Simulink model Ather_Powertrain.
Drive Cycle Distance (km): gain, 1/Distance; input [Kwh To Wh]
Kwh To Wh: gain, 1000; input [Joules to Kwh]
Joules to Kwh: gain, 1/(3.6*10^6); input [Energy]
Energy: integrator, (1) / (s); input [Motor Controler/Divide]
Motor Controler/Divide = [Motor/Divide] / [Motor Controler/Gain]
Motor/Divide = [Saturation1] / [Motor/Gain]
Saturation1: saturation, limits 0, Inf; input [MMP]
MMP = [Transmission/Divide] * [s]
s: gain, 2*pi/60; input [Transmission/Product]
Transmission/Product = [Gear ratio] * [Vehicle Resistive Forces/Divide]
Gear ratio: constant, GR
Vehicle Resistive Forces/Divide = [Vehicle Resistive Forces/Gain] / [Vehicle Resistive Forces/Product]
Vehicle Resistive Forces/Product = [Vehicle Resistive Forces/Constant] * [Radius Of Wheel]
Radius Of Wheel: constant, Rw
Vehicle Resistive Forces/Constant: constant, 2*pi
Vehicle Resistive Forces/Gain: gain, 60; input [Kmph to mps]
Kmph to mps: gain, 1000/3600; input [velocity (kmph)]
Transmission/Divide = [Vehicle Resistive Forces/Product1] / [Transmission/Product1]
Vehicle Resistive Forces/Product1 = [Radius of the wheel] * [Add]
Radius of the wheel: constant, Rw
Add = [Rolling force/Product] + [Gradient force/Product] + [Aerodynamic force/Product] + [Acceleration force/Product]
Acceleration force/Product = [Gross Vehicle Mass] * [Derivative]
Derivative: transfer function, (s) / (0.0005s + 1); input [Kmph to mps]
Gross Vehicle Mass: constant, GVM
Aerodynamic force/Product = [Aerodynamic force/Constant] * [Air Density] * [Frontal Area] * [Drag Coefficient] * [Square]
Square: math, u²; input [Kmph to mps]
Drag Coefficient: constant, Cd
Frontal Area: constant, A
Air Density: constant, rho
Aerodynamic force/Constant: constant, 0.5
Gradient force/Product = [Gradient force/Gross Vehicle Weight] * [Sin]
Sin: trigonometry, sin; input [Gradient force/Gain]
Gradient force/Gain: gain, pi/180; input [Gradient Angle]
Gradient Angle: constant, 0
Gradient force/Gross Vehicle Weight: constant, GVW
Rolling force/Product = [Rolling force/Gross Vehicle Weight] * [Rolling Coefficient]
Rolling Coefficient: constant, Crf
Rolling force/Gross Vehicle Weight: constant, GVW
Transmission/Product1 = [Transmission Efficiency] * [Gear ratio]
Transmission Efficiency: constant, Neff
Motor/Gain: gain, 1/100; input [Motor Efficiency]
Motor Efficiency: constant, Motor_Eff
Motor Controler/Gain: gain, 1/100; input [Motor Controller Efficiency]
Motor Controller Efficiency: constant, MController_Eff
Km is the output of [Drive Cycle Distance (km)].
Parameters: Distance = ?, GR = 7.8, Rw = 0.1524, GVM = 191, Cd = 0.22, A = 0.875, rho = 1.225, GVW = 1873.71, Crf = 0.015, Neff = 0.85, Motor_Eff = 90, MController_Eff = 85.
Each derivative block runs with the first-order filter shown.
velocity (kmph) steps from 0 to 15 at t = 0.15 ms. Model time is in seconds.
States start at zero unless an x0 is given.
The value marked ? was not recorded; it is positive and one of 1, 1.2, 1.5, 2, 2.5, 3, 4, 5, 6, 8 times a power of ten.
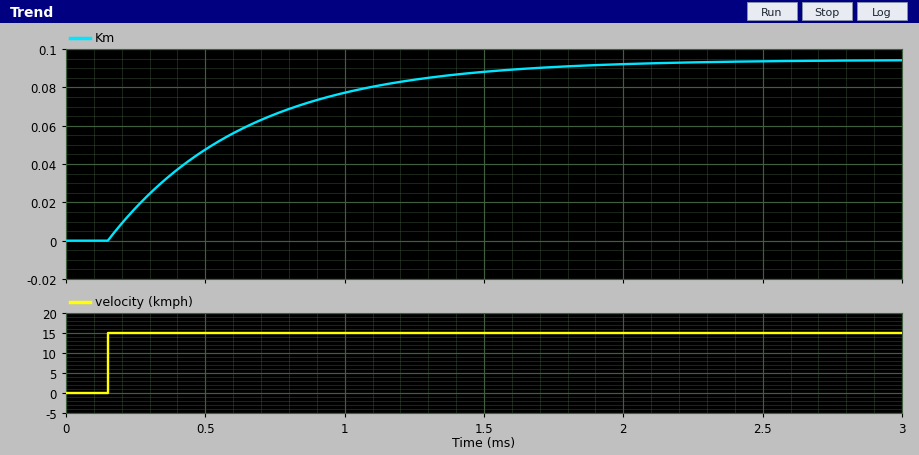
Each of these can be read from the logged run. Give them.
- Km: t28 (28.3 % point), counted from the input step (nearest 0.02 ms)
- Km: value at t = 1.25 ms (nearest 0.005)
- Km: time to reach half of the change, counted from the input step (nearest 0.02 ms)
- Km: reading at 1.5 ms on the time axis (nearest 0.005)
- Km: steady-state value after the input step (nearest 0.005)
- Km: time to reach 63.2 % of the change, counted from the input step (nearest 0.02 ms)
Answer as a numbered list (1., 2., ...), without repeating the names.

1. 0.16 ms
2. 0.085
3. 0.34 ms
4. 0.090
5. 0.095
6. 0.50 ms
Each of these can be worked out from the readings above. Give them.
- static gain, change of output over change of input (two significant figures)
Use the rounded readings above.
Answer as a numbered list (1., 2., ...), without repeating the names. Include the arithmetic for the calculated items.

1. (0.095 - 0) / (15 - 0) = 0.0063
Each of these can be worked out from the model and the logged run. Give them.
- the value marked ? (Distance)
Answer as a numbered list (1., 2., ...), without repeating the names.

1. 15
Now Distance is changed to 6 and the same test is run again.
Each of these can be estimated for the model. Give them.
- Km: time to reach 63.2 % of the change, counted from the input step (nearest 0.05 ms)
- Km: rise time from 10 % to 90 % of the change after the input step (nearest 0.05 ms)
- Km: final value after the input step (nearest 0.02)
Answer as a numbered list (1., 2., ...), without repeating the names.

1. 0.50 ms
2. 1.10 ms
3. 0.24
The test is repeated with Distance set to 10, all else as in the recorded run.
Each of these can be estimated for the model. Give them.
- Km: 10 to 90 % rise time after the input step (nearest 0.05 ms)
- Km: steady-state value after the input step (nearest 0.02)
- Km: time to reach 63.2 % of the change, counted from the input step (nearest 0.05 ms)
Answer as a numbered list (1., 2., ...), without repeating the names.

1. 1.10 ms
2. 0.14
3. 0.50 ms
